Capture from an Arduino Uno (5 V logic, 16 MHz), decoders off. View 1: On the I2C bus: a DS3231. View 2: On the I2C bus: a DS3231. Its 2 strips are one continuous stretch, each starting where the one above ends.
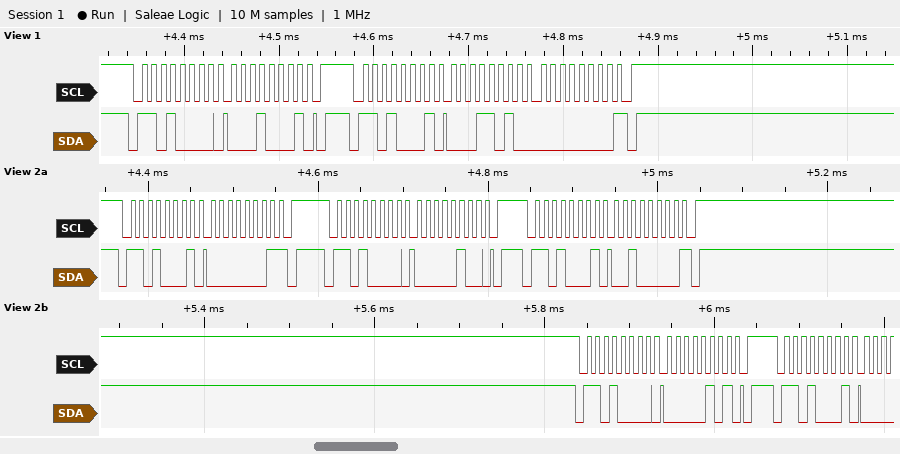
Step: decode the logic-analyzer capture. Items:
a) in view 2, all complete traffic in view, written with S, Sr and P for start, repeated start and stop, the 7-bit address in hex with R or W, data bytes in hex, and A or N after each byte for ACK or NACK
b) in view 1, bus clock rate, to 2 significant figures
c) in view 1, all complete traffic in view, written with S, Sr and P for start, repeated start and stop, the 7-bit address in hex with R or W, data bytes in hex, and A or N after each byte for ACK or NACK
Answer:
S 68R A 01 N P S 68W A 04 A P S 68R A 20 N P S 68W A 05 A P S 68R A
100 kHz
S 68W A 11 A P S 68R A 1A A 00 N P
